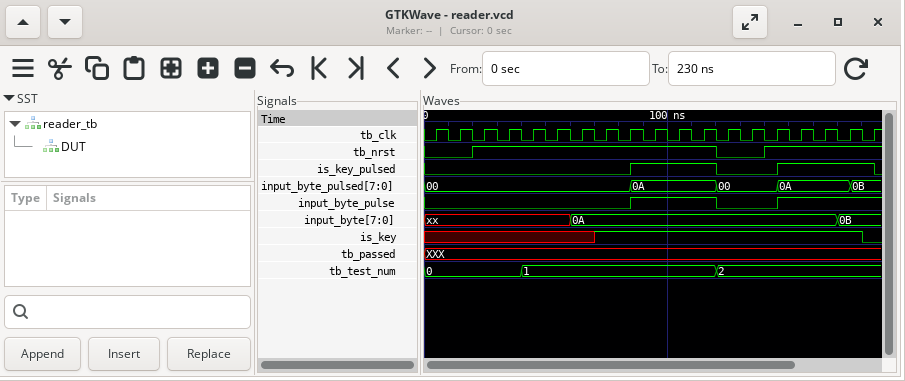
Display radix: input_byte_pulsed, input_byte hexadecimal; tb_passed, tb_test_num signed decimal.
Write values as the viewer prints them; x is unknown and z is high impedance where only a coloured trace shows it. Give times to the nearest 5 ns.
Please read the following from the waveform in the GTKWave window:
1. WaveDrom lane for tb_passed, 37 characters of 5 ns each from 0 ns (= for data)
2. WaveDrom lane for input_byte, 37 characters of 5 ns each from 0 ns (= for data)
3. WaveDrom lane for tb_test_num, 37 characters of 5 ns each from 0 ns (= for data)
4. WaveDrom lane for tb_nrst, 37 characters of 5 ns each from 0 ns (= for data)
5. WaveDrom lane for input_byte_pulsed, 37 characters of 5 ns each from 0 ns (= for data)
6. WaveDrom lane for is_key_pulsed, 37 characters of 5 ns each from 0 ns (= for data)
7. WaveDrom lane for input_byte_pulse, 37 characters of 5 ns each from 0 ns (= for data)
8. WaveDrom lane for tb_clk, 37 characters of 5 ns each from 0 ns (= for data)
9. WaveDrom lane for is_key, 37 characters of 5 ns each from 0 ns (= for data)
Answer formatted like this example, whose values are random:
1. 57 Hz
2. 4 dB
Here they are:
1. {name: 'tb_passed', wave: 'x....................................'}
2. {name: 'input_byte', wave: 'x...........=.....................=..', data: '0A 0B'}
3. {name: 'tb_test_num', wave: '=.......=...............=............', data: '0 1 2'}
4. {name: 'tb_nrst', wave: '0...1...................0...1........'}
5. {name: 'input_byte_pulsed', wave: '=................=......=....=.....=.', data: '00 0A 00 0A 0B'}
6. {name: 'is_key_pulsed', wave: '0................1......0....1.......'}
7. {name: 'input_byte_pulse', wave: '0................1......0....1.......'}
8. {name: 'tb_clk', wave: '0101010101010101010101010101010101010'}
9. {name: 'is_key', wave: 'x.............1.....................0'}
